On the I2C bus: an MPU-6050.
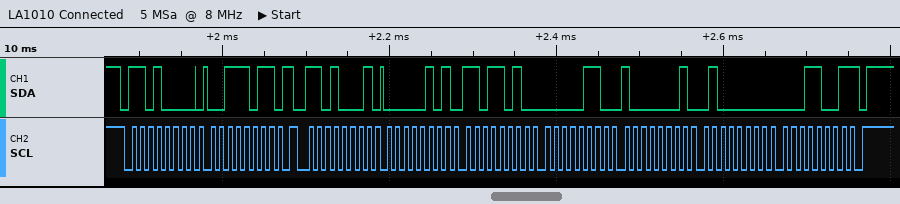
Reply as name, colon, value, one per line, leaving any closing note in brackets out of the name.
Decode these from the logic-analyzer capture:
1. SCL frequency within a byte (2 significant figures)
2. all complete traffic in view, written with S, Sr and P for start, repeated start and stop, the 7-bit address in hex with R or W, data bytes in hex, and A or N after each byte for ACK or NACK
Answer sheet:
SCL frequency within a byte: 100 kHz
all complete traffic in view, written with S, Sr and P for start, repeated start and stop, the 7-bit address in hex with R or W, data bytes in hex, and A or N after each byte for ACK or NACK: S 68W A 3B A Sr 68R A 05 A DA A 06 A 81 A 40 A 19 N P
